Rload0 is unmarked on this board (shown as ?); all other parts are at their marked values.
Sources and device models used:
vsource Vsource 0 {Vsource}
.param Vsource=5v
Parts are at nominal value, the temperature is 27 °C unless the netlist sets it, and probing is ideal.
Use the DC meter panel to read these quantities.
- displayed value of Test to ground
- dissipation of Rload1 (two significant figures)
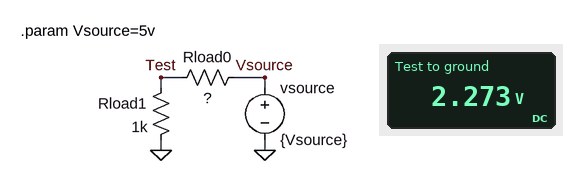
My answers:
2.273 V
5.2 mW
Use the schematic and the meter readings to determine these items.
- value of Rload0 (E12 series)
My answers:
1.2 kΩ
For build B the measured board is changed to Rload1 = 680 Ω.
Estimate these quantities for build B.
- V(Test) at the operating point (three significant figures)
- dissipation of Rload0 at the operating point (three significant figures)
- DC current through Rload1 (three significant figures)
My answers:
1.81 V
8.49 mW
2.66 mA
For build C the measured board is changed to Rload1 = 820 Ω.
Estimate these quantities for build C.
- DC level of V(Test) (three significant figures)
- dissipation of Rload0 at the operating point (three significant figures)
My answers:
2.03 V
7.35 mW
